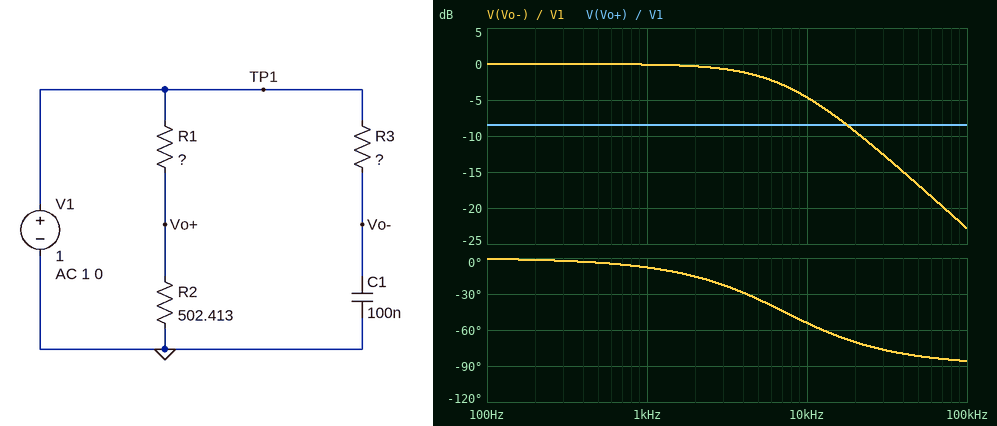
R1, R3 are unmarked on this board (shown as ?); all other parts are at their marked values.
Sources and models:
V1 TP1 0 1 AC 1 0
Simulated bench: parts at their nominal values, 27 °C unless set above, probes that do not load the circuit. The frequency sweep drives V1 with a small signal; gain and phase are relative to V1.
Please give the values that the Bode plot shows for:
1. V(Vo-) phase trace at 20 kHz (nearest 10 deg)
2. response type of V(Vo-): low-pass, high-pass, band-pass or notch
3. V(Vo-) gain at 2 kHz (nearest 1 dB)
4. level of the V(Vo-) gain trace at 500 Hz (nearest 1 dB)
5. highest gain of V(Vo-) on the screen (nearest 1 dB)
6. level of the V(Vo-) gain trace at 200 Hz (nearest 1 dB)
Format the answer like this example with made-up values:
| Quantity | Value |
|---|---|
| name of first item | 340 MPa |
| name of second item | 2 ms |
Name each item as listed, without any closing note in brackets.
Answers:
| Quantity | Value |
|---|---|
| V(Vo-) phase trace at 20 kHz | -70 deg |
| response type of V(Vo-): low-pass, high-pass, band-pass or notch | low-pass |
| V(Vo-) gain at 2 kHz | 0 dB |
| level of the V(Vo-) gain trace at 500 Hz | 0 dB |
| highest gain of V(Vo-) on the screen | 0 dB |
| level of the V(Vo-) gain trace at 200 Hz | 0 dB |
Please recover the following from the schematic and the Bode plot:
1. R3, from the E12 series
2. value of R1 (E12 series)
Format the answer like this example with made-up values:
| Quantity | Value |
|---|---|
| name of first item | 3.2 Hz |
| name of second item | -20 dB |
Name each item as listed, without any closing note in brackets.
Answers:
| Quantity | Value |
|---|---|
| R3, from the E12 series | 220 Ω |
| value of R1 | 820 Ω |
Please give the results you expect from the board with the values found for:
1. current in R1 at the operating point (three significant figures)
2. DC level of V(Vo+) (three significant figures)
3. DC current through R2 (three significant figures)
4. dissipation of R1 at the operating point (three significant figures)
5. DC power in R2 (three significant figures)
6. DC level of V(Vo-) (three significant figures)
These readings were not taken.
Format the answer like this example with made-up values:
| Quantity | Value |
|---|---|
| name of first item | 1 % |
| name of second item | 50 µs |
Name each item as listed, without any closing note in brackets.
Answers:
| Quantity | Value |
|---|---|
| current in R1 at the operating point | 756 µA |
| DC level of V(Vo+) | 380 mV |
| DC current through R2 | 756 µA |
| dissipation of R1 at the operating point | 469 µW |
| DC power in R2 | 287 µW |
| DC level of V(Vo-) | 1.00 V |
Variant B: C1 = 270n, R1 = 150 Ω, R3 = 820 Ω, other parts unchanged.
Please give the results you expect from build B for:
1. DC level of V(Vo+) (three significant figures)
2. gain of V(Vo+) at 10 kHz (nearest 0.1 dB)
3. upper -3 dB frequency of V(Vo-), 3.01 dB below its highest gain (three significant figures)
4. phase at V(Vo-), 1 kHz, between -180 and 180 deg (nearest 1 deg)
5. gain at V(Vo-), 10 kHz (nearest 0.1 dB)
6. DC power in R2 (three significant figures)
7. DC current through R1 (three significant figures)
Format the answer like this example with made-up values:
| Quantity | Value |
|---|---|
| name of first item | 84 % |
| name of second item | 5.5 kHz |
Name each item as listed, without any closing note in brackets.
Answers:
| Quantity | Value |
|---|---|
| DC level of V(Vo+) | 770 mV |
| gain of V(Vo+) at 10 kHz | -2.3 dB |
| upper -3 dB frequency of V(Vo-), 3.01 dB below its highest gain | 719 Hz |
| phase at V(Vo-), 1 kHz, between -180 and 180 deg | -54 deg |
| gain at V(Vo-), 10 kHz | -22.9 dB |
| DC power in R2 | 1.18 mW |
| DC current through R1 | 1.53 mA |
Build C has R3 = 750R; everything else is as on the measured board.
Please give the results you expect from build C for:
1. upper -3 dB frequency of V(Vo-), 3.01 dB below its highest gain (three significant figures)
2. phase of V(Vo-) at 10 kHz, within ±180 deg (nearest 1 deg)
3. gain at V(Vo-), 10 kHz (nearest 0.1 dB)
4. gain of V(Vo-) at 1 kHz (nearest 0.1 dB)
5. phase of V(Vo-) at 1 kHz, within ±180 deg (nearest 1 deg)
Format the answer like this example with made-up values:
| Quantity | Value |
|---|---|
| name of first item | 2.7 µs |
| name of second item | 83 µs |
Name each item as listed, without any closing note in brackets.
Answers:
| Quantity | Value |
|---|---|
| upper -3 dB frequency of V(Vo-), 3.01 dB below its highest gain | 2.12 kHz |
| phase of V(Vo-) at 10 kHz, within ±180 deg | -78 deg |
| gain at V(Vo-), 10 kHz | -13.7 dB |
| gain of V(Vo-) at 1 kHz | -0.9 dB |
| phase of V(Vo-) at 1 kHz, within ±180 deg | -25 deg |
